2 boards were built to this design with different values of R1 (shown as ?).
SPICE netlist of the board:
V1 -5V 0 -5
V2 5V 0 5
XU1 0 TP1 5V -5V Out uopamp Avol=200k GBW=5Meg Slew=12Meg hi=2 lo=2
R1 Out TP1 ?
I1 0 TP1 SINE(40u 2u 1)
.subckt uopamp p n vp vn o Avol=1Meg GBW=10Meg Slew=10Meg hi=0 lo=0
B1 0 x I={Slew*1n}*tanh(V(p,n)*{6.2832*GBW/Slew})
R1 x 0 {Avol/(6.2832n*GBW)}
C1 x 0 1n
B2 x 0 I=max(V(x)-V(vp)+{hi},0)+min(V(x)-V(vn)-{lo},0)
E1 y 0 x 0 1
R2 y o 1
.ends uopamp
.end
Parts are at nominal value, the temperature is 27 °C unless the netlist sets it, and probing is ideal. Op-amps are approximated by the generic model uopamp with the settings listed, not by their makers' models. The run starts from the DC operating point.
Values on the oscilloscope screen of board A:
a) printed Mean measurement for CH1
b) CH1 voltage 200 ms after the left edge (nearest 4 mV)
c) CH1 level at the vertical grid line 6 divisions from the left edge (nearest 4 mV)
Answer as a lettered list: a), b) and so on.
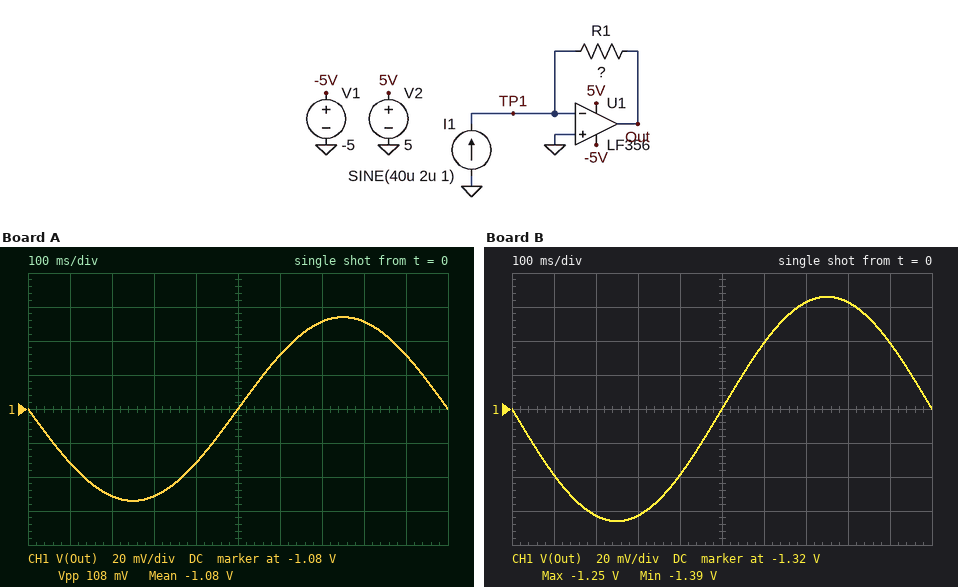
a) -1.08 V
b) -1.132 V
c) -1.048 V
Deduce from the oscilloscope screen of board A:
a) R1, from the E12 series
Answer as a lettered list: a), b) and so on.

a) 27 kΩ
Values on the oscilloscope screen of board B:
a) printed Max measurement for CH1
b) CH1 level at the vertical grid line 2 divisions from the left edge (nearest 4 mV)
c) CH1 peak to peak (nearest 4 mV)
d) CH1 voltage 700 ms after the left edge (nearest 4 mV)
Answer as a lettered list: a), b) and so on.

a) -1.25 V
b) -1.384 V
c) 132 mV
d) -1.256 V
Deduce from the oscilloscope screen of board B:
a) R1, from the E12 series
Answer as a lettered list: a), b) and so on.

a) 33 kΩ
